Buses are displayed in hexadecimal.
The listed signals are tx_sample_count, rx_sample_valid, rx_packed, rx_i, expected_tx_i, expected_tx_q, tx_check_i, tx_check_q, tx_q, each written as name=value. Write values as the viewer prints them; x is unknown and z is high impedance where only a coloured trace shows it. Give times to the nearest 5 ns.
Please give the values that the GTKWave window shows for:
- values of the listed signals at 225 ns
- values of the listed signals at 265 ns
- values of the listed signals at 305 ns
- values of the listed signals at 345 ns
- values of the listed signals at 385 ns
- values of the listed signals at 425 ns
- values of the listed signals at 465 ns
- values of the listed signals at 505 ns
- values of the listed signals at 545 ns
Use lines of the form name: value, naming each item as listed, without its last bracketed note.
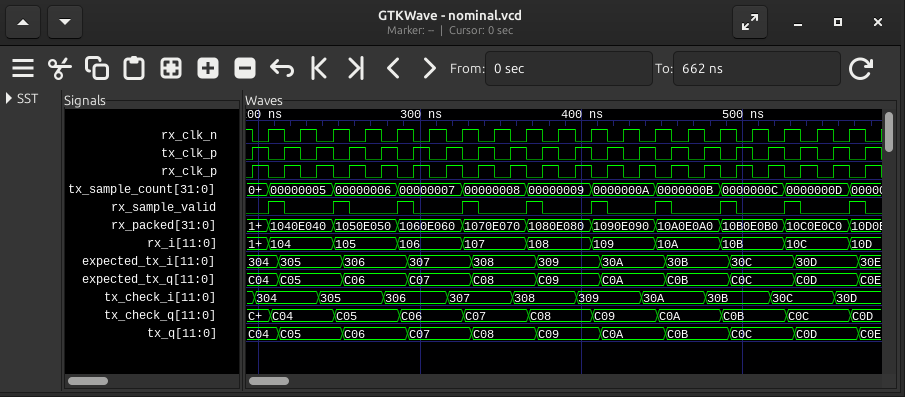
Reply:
values of the listed signals at 225 ns: tx_sample_count=00000005, rx_sample_valid=0, rx_packed=1040E040, rx_i=104, expected_tx_i=305, expected_tx_q=C05, tx_check_i=304, tx_check_q=C04, tx_q=C05
values of the listed signals at 265 ns: tx_sample_count=00000006, rx_sample_valid=0, rx_packed=1050E050, rx_i=105, expected_tx_i=306, expected_tx_q=C06, tx_check_i=305, tx_check_q=C05, tx_q=C06
values of the listed signals at 305 ns: tx_sample_count=00000007, rx_sample_valid=0, rx_packed=1060E060, rx_i=106, expected_tx_i=307, expected_tx_q=C07, tx_check_i=306, tx_check_q=C06, tx_q=C07
values of the listed signals at 345 ns: tx_sample_count=00000008, rx_sample_valid=0, rx_packed=1070E070, rx_i=107, expected_tx_i=308, expected_tx_q=C08, tx_check_i=307, tx_check_q=C07, tx_q=C08
values of the listed signals at 385 ns: tx_sample_count=00000009, rx_sample_valid=0, rx_packed=1080E080, rx_i=108, expected_tx_i=309, expected_tx_q=C09, tx_check_i=308, tx_check_q=C08, tx_q=C09
values of the listed signals at 425 ns: tx_sample_count=0000000A, rx_sample_valid=0, rx_packed=1090E090, rx_i=109, expected_tx_i=30A, expected_tx_q=C0A, tx_check_i=309, tx_check_q=C09, tx_q=C0A
values of the listed signals at 465 ns: tx_sample_count=0000000B, rx_sample_valid=0, rx_packed=10A0E0A0, rx_i=10A, expected_tx_i=30B, expected_tx_q=C0B, tx_check_i=30A, tx_check_q=C0A, tx_q=C0B
values of the listed signals at 505 ns: tx_sample_count=0000000C, rx_sample_valid=0, rx_packed=10B0E0B0, rx_i=10B, expected_tx_i=30C, expected_tx_q=C0C, tx_check_i=30B, tx_check_q=C0B, tx_q=C0C
values of the listed signals at 545 ns: tx_sample_count=0000000D, rx_sample_valid=0, rx_packed=10C0E0C0, rx_i=10C, expected_tx_i=30D, expected_tx_q=C0D, tx_check_i=30C, tx_check_q=C0C, tx_q=C0D
